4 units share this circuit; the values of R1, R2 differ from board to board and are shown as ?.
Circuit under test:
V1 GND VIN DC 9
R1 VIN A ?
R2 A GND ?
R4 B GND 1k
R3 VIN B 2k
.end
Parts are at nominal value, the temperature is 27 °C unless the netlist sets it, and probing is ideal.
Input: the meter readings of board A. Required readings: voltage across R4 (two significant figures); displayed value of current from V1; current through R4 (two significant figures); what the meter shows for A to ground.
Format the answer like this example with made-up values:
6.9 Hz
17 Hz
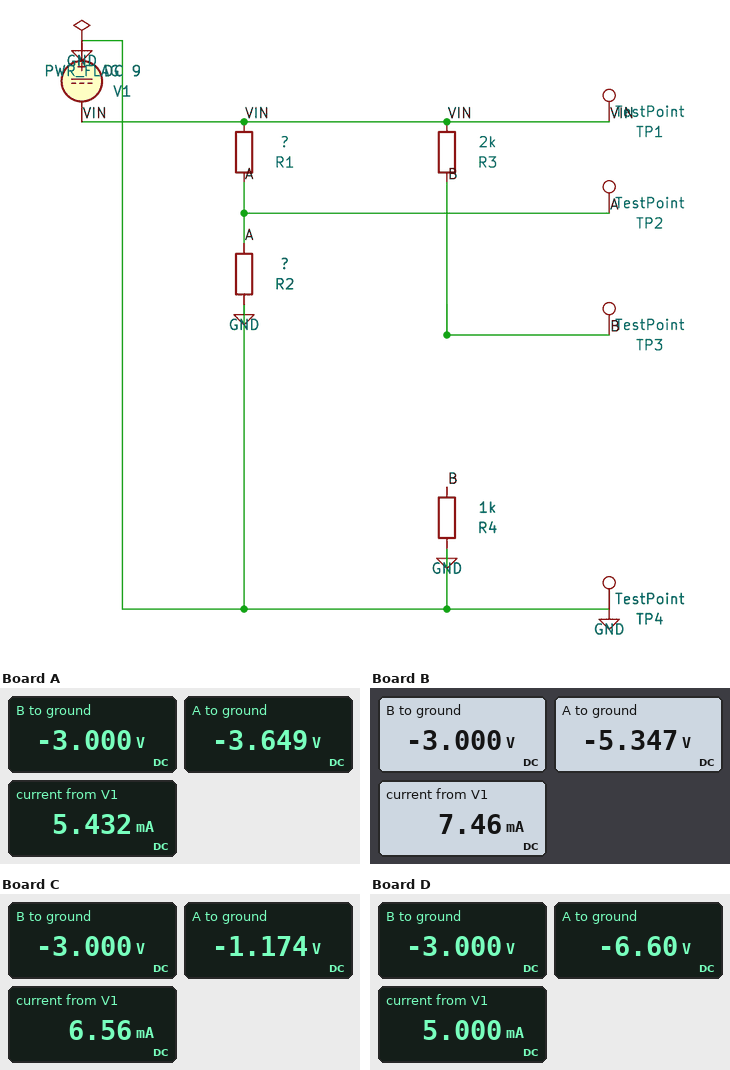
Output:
3.0 V
5.432 mA
3.0 mA
-3.649 V
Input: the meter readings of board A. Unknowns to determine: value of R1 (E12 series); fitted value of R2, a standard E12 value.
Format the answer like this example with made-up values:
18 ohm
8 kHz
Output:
2.2 kΩ
1.5 kΩ
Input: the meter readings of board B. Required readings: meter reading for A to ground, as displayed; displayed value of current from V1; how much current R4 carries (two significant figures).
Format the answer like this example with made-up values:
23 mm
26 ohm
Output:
-5.347 V
7.46 mA
3.0 mA
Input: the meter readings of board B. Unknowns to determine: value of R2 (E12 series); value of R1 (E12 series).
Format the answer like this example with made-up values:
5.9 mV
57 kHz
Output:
1.2 kΩ
820 Ω
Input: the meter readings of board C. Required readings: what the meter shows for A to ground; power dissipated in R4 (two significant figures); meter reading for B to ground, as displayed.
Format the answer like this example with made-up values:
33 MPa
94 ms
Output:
-1.174 V
9.0 mW
-3.000 V
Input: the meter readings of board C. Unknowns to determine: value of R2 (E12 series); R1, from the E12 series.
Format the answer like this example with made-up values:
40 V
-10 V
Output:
330 Ω
2.2 kΩ
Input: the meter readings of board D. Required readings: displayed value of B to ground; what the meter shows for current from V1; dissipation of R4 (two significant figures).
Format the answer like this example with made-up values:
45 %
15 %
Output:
-3.000 V
5.000 mA
9.0 mW
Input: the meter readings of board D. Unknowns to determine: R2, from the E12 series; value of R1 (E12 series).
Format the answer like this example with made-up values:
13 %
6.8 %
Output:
3.3 kΩ
1.2 kΩ
